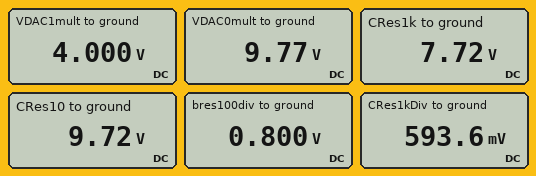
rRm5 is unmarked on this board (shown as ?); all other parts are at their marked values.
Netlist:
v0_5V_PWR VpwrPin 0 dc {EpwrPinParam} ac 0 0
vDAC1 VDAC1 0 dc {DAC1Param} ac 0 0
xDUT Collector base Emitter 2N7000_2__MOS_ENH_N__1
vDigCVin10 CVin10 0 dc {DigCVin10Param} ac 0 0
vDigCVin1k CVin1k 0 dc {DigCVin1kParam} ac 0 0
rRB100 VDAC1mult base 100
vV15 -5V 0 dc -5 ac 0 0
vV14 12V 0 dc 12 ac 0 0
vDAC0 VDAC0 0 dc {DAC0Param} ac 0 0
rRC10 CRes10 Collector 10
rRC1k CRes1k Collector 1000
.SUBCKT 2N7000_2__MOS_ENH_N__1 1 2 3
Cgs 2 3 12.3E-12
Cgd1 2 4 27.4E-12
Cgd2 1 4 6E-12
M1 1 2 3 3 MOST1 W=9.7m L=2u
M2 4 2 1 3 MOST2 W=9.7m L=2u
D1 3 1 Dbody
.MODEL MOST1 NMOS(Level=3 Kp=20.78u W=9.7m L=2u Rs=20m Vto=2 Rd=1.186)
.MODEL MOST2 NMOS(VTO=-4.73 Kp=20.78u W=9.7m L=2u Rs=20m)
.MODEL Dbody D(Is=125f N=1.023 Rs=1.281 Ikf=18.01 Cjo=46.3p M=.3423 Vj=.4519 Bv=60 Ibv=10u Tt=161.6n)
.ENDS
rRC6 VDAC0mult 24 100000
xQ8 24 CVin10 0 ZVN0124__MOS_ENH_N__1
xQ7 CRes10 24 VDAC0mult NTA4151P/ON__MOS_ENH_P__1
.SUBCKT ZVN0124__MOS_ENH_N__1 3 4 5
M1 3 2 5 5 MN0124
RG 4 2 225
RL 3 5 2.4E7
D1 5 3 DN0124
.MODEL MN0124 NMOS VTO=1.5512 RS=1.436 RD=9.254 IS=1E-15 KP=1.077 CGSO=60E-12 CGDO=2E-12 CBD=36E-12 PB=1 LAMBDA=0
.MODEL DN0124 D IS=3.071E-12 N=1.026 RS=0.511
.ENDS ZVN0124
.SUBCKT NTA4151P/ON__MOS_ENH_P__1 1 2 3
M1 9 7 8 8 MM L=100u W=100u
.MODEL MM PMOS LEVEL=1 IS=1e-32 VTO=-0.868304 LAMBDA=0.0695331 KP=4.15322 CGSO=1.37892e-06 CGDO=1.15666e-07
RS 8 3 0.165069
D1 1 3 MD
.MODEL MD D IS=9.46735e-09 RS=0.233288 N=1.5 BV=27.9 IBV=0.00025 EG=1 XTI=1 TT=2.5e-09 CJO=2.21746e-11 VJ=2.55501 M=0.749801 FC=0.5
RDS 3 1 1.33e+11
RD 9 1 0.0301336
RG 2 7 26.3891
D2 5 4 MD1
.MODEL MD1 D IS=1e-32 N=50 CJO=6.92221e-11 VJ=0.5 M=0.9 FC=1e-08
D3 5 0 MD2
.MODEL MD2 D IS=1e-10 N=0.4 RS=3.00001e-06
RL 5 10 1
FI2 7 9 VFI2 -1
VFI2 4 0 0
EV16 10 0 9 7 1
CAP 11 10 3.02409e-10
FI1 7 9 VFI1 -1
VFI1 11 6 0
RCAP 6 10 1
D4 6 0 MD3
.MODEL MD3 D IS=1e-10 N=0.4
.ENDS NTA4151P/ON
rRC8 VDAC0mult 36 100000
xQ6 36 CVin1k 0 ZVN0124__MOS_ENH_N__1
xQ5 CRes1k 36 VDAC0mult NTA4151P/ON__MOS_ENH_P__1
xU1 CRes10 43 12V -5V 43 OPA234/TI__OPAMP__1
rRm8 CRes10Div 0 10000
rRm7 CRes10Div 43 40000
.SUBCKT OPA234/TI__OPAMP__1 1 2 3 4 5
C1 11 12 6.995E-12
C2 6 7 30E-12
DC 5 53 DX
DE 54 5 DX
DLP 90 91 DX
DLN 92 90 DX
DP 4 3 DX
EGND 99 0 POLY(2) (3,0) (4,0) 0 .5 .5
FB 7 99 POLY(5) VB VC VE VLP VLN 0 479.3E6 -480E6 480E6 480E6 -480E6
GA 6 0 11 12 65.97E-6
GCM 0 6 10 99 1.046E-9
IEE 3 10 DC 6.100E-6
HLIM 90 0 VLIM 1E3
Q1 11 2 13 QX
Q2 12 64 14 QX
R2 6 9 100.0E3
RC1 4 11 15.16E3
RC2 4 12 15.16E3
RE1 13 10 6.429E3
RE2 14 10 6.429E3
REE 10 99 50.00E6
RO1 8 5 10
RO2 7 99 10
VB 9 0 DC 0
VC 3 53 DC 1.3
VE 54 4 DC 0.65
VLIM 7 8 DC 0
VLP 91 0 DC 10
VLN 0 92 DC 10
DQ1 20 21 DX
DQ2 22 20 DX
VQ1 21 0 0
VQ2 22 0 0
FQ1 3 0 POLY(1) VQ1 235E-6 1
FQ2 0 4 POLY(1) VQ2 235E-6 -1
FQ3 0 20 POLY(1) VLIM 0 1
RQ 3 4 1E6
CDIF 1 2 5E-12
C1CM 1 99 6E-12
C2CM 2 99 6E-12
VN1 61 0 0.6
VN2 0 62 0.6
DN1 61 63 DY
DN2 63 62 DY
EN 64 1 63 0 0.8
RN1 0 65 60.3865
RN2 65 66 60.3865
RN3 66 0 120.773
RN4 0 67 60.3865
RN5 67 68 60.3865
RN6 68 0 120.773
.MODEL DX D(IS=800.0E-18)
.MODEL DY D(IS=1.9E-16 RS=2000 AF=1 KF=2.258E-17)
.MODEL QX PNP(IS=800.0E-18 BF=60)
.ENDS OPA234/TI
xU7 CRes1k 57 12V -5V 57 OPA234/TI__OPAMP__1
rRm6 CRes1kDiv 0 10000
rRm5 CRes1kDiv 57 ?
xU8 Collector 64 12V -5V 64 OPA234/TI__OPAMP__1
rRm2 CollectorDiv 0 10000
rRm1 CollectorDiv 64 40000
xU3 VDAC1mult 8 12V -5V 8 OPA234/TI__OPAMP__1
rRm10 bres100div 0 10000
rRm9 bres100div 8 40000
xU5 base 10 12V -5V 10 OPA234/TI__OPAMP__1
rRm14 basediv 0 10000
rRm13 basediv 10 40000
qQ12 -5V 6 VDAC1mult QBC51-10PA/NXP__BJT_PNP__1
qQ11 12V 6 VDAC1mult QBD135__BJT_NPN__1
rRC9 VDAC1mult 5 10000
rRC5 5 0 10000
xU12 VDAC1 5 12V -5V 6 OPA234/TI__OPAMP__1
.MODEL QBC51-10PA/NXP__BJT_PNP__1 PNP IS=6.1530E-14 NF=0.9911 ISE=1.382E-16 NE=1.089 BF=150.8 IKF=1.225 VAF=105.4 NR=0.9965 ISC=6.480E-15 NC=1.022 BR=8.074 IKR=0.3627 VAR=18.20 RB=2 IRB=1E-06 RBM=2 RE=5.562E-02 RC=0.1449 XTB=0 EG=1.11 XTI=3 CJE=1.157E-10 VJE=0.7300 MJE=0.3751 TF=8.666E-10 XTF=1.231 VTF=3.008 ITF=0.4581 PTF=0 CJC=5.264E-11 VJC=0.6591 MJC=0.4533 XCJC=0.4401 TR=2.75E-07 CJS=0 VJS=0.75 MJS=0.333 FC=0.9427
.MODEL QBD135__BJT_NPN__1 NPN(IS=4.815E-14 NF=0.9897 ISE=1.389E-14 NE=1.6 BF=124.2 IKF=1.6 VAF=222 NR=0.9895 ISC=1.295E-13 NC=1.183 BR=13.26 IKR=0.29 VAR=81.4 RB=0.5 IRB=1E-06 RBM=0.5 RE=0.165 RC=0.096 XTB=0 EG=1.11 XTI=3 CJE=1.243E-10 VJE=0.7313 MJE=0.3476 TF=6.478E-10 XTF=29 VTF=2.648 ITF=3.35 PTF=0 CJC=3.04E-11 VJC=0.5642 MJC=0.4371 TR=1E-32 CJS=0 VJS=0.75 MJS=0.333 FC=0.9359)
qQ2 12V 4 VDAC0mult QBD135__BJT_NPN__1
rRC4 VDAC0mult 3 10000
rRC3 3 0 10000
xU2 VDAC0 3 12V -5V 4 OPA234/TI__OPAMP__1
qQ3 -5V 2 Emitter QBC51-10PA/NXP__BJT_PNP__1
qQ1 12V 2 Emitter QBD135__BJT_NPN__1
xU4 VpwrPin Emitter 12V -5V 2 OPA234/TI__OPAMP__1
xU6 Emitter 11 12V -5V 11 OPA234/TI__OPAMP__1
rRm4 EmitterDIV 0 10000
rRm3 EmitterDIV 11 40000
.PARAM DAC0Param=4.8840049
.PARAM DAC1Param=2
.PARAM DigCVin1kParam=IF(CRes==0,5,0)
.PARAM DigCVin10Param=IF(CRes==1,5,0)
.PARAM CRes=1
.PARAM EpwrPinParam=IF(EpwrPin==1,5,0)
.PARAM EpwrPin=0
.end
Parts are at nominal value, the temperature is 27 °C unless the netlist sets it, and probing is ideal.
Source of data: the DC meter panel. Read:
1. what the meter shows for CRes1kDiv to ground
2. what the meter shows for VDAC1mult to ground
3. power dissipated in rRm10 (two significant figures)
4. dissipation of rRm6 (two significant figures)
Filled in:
593.6 mV
4.000 V
64 µW
35 µW
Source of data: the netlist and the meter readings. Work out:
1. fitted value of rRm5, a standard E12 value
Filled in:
120 kΩ
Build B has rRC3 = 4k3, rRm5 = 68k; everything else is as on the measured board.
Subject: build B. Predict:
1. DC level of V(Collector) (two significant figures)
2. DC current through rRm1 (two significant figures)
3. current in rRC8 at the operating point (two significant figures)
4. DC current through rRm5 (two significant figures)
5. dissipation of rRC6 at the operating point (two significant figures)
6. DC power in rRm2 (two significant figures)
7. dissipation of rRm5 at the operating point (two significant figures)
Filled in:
8.5 V
170 µA
440 nA
110 µA
1.1 mW
290 µW
800 µW
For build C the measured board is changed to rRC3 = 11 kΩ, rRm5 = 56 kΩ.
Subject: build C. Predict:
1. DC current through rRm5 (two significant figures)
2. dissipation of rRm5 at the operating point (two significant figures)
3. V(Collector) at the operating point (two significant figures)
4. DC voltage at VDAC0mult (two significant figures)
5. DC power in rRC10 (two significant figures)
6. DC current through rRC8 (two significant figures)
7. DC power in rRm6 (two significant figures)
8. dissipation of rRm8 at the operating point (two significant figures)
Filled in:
110 µA
680 µW
7.3 V
9.3 V
400 mW
390 nA
120 µW
340 µW
